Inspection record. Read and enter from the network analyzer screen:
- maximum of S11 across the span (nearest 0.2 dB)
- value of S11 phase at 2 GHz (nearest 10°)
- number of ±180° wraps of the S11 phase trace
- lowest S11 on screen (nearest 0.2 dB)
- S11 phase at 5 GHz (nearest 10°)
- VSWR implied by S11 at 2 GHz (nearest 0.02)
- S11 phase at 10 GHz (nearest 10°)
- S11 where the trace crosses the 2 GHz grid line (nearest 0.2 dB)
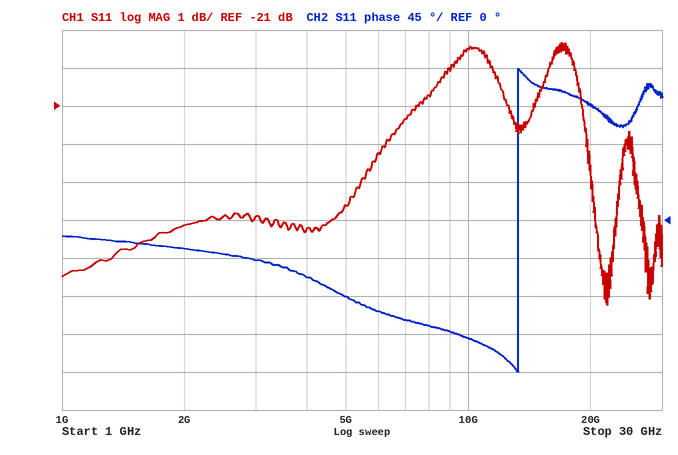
-19.4 dB
-30°
1
-26.2 dB
-90°
1.14
-140°
-24.2 dB
